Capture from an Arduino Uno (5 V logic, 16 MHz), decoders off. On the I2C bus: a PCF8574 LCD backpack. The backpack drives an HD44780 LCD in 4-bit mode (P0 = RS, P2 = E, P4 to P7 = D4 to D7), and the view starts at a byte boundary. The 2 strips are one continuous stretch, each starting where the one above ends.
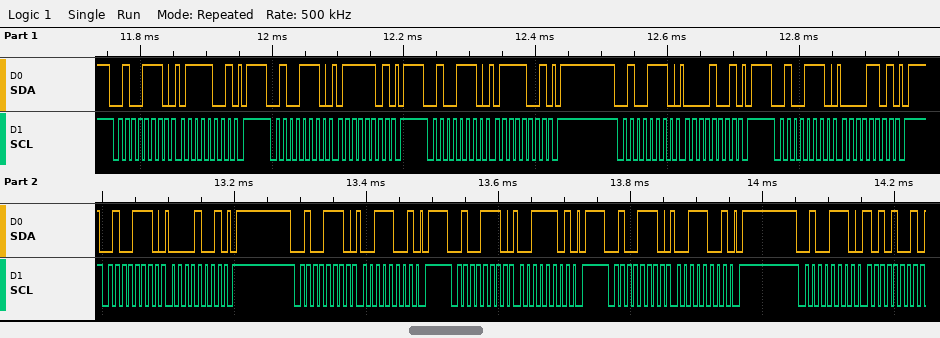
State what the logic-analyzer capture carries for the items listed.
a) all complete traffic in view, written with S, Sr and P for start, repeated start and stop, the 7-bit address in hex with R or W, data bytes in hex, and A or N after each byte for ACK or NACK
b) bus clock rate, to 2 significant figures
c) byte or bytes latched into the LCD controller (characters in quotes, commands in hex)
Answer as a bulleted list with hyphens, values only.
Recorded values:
- S 27W A 79 A P S 27W A 7D A P S 27W A 79 A P S 27W A 09 A P S 27W A 0D A P S 27W A 09 A P S 27W A 39 A P S 27W A 3D A P S 27W A 39 A P S 27W A A9 A
- 100 kHz
- 'p'
